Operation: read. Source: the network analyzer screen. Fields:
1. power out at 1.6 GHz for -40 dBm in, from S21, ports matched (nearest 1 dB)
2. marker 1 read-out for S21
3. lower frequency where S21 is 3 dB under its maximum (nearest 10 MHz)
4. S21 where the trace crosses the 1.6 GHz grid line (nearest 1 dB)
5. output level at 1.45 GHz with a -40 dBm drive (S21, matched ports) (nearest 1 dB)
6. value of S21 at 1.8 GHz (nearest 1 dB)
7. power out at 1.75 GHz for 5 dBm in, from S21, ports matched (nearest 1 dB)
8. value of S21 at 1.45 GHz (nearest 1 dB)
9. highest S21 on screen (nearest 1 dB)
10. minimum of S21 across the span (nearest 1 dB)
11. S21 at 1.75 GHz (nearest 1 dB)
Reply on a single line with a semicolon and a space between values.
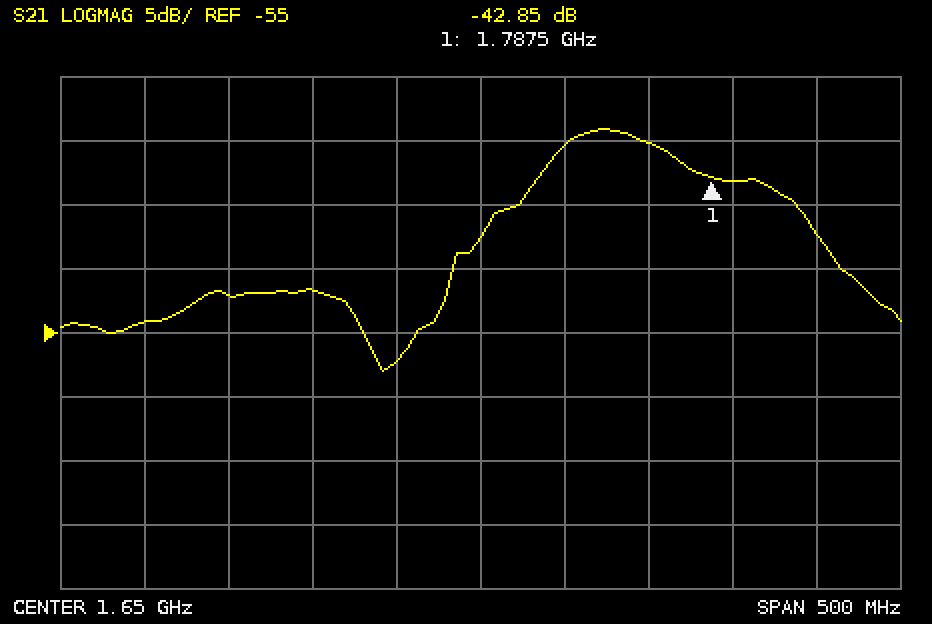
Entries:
-97 dBm; -42.85 dB; 1.69 GHz; -57 dB; -94 dBm; -43 dB; -35 dBm; -54 dB; -39 dB; -58 dB; -40 dB
